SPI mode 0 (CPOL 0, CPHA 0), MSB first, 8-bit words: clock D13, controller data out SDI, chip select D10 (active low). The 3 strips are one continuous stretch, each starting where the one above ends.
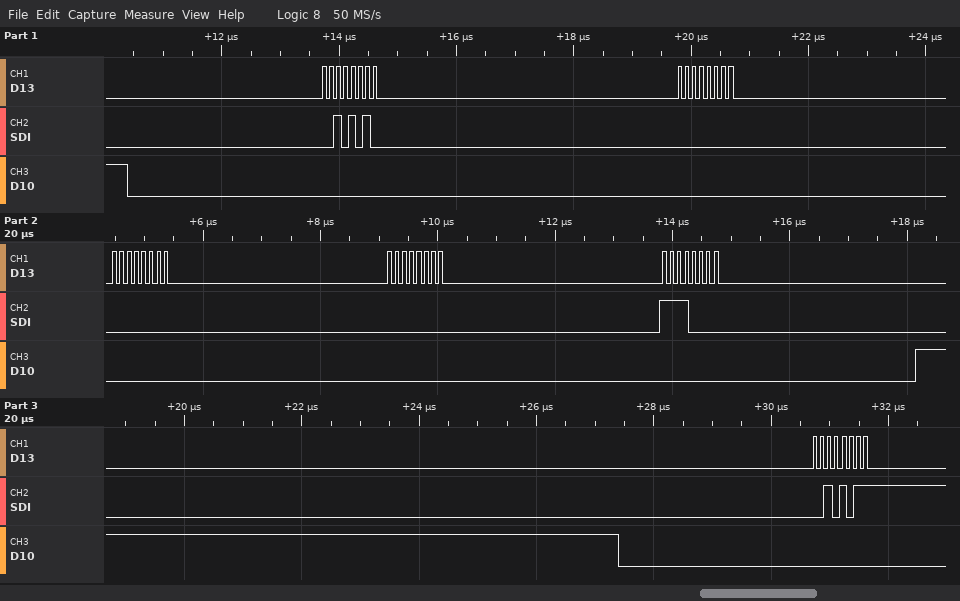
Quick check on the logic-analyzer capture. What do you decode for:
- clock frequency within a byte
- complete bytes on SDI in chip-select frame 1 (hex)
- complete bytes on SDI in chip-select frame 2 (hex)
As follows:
8 MHz
2A 00 00 00 F0
2B
